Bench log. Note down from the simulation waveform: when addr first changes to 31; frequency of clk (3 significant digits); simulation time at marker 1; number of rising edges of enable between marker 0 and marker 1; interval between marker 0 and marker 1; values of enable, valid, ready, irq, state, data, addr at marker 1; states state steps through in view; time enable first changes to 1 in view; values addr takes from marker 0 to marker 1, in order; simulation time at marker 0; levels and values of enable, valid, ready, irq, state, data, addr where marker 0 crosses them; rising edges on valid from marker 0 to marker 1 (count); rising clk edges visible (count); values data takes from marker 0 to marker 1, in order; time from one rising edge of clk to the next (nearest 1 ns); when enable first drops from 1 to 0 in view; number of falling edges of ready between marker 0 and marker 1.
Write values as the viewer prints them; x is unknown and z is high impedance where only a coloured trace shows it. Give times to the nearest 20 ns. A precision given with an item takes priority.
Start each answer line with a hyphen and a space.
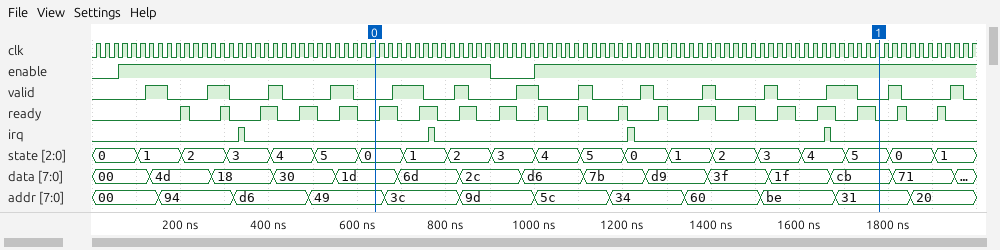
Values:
- 1680 ns
- 50.0 MHz
- 1780 ns
- 1
- 1140 ns
- enable=1, valid=0, ready=0, irq=0, state=5, data=cb, addr=31
- 0, 1, 2, 3, 4, 5, 0, 1, 2, 3, 4, 5, 0, 1, 2, 3, 4, 5, 0, 1
- 60 ns
- 49, 3c, 9d, 5c, 34, 60, be, 31
- 640 ns
- enable=1, valid=0, ready=0, irq=0, state=0, data=1d, addr=49
- 8
- 100
- 1d, 6d, 2c, d6, 7b, d9, 3f, 1f, cb
- 20 ns
- 900 ns
- 13
